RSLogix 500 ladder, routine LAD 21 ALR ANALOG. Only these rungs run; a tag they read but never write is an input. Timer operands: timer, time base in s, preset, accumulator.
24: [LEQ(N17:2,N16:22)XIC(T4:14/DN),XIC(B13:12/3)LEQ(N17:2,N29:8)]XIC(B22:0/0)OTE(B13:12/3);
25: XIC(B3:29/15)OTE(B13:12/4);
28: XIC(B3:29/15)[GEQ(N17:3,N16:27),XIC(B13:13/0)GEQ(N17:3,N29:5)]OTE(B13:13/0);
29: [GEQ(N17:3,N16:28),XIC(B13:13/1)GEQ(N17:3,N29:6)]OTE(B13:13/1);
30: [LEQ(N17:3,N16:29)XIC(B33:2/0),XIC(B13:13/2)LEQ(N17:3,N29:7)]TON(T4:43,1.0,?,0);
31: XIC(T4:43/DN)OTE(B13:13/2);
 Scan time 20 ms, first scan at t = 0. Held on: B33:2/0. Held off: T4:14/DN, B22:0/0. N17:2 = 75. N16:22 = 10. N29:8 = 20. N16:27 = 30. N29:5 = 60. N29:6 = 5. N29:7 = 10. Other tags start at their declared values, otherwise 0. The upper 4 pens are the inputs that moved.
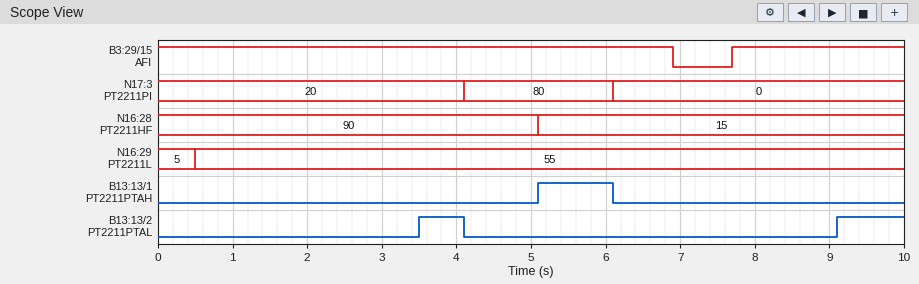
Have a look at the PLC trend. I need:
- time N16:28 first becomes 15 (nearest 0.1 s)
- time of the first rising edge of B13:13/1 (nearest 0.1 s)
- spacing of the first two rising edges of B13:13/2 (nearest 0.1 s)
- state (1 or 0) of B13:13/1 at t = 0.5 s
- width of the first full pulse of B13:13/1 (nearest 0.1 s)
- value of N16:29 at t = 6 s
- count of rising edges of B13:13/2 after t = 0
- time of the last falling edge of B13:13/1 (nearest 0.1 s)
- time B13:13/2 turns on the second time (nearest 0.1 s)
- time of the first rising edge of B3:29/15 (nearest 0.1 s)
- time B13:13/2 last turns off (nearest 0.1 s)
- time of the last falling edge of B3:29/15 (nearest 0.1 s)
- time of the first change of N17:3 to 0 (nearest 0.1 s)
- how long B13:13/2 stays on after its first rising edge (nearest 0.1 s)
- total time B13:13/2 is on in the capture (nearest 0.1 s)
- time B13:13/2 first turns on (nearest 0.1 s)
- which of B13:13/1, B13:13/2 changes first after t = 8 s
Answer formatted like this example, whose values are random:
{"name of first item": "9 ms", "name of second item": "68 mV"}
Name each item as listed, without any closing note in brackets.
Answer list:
{"time N16:28 first becomes 15": "5.1 s", "time of the first rising edge of B13:13/1": "5.1 s", "spacing of the first two rising edges of B13:13/2": "5.6 s", "state (1 or 0) of B13:13/1 at t = 0.5 s": "0", "width of the first full pulse of B13:13/1": "1.0 s", "value of N16:29 at t = 6 s": "55", "count of rising edges of B13:13/2 after t = 0": "2", "time of the last falling edge of B13:13/1": "6.1 s", "time B13:13/2 turns on the second time": "9.1 s", "time of the first rising edge of B3:29/15": "7.7 s", "time B13:13/2 last turns off": "4.1 s", "time of the last falling edge of B3:29/15": "6.9 s", "time of the first change of N17:3 to 0": "6.1 s", "how long B13:13/2 stays on after its first rising edge": "0.6 s", "total time B13:13/2 is on in the capture": "1.5 s", "time B13:13/2 first turns on": "3.5 s", "which of B13:13/1, B13:13/2 changes first after t = 8 s": "B13:13/2"}
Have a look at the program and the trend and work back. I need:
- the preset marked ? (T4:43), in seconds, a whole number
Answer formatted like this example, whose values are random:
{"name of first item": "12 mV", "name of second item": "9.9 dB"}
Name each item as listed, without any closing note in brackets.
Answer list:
{"the preset marked ? (T4:43), in seconds, a whole number": "3 s"}
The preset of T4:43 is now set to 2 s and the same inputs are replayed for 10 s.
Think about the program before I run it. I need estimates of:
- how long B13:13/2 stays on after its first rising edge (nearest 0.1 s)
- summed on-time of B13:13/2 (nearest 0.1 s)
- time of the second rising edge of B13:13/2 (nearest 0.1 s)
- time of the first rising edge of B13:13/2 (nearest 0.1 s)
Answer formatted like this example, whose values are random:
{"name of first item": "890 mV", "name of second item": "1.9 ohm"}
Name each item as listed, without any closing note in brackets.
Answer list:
{"how long B13:13/2 stays on after its first rising edge": "1.6 s", "summed on-time of B13:13/2": "3.5 s", "time of the second rising edge of B13:13/2": "8.1 s", "time of the first rising edge of B13:13/2": "2.5 s"}
